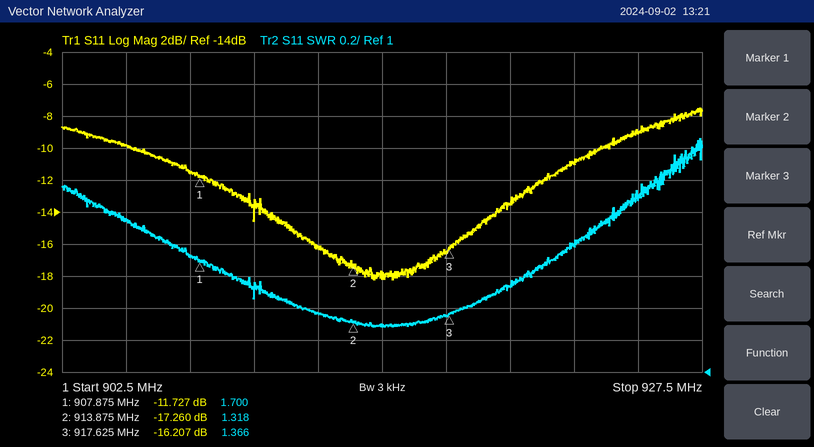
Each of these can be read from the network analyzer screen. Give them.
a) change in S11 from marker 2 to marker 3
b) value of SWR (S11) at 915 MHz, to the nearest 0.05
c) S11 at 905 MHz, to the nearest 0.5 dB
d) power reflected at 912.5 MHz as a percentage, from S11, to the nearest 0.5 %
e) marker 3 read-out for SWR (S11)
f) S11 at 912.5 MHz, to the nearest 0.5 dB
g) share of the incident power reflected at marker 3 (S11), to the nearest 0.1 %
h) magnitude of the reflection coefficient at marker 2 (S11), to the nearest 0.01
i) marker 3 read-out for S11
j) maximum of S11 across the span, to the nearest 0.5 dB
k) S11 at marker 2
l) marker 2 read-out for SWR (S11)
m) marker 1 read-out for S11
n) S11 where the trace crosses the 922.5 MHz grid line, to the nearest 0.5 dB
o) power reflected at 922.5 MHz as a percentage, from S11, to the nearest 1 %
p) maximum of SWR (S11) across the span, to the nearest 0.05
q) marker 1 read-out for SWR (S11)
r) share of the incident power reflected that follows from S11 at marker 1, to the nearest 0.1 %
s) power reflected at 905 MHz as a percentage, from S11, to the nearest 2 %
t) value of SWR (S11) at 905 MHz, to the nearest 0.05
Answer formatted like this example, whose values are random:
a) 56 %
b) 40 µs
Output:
a) 1.053 dB
b) 1.30
c) -10.0 dB
d) 2.5 %
e) 1.366
f) -16.0 dB
g) 2.4 %
h) 0.14
i) -16.207 dB
j) -7.5 dB
k) -17.260 dB
l) 1.318
m) -11.727 dB
n) -11.0 dB
o) 8 %
p) 2.45
q) 1.700
r) 6.7 %
s) 10 %
t) 1.95
